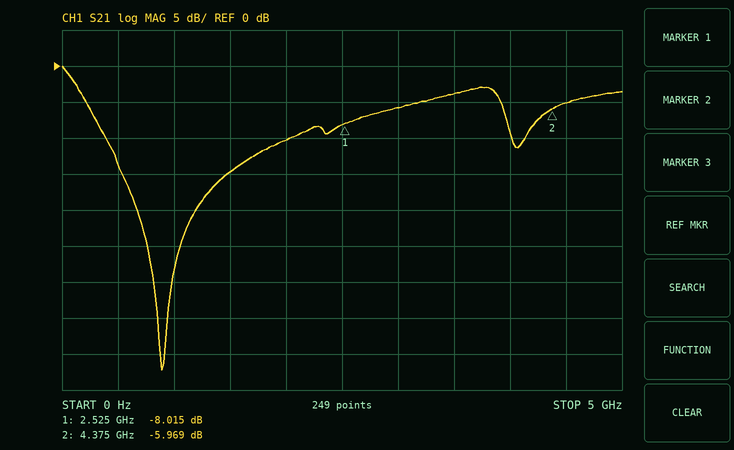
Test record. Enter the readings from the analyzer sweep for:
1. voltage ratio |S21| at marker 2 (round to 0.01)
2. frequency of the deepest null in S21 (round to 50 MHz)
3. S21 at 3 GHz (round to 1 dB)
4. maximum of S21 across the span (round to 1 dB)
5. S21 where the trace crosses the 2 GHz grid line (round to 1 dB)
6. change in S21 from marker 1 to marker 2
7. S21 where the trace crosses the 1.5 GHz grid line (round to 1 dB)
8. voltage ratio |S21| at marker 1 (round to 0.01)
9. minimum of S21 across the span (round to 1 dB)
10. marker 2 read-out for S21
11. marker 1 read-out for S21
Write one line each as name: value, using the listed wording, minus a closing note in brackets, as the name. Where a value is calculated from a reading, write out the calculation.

voltage ratio |S21| at marker 2: 10^(-5.969/20) ≈ 0.50
frequency of the deepest null in S21: 900 MHz
S21 at 3 GHz: -6 dB
maximum of S21 across the span: 0 dB
S21 where the trace crosses the 2 GHz grid line: -10 dB
change in S21 from marker 1 to marker 2: -5.969 − (-8.015) = 2.046 dB
S21 where the trace crosses the 1.5 GHz grid line: -15 dB
voltage ratio |S21| at marker 1: 10^(-8.015/20) ≈ 0.40
minimum of S21 across the span: -42 dB
marker 2 read-out for S21: -5.969 dB
marker 1 read-out for S21: -8.015 dB
